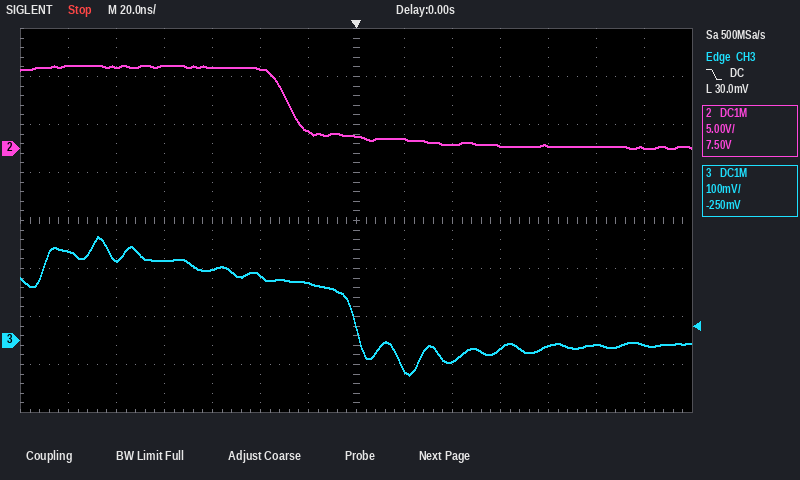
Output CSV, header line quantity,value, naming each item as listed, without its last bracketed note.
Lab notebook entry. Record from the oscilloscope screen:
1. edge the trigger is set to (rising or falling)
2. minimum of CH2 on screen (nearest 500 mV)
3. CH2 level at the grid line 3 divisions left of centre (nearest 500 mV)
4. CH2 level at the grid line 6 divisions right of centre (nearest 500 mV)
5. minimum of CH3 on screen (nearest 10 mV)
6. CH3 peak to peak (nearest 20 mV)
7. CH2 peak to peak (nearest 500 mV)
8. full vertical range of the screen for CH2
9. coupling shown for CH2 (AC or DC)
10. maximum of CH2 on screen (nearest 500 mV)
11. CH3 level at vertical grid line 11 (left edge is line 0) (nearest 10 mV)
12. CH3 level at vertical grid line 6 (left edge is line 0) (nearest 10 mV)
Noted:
quantity,value
edge the trigger is set to,falling
minimum of CH2 on screen,0.0 V
CH2 level at the grid line 3 divisions left of centre,8.5 V
CH2 level at the grid line 6 divisions right of centre,0.0 V
minimum of CH3 on screen,-70 mV
CH3 peak to peak,280 mV
CH2 peak to peak,8.5 V
full vertical range of the screen for CH2,40 V
coupling shown for CH2,DC
maximum of CH2 on screen,8.5 V
CH3 level at vertical grid line 11 (left edge is line 0),-10 mV
CH3 level at vertical grid line 6 (left edge is line 0),120 mV
